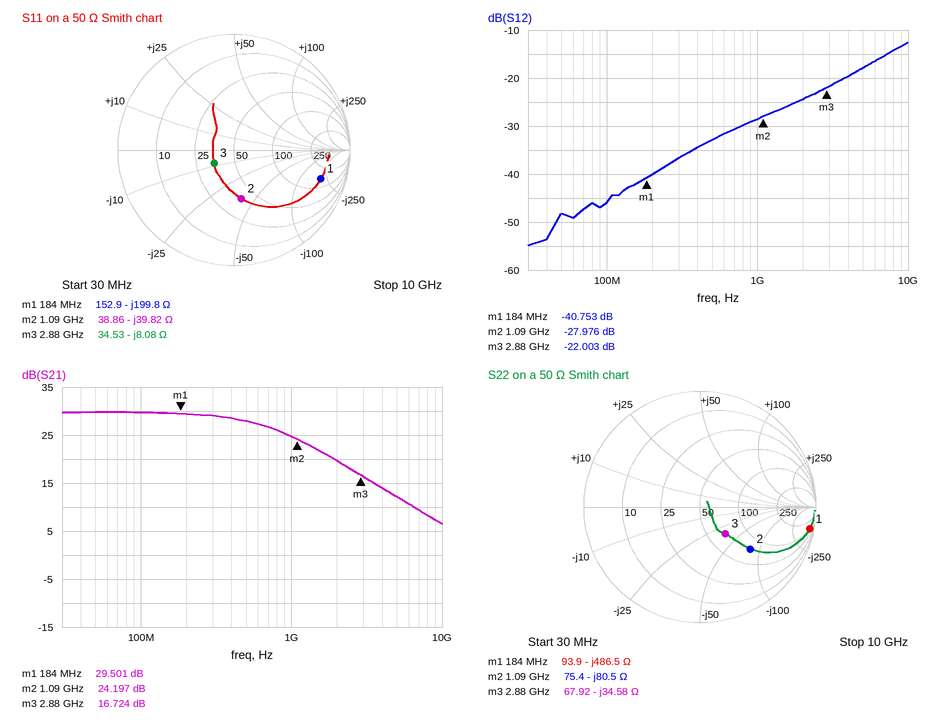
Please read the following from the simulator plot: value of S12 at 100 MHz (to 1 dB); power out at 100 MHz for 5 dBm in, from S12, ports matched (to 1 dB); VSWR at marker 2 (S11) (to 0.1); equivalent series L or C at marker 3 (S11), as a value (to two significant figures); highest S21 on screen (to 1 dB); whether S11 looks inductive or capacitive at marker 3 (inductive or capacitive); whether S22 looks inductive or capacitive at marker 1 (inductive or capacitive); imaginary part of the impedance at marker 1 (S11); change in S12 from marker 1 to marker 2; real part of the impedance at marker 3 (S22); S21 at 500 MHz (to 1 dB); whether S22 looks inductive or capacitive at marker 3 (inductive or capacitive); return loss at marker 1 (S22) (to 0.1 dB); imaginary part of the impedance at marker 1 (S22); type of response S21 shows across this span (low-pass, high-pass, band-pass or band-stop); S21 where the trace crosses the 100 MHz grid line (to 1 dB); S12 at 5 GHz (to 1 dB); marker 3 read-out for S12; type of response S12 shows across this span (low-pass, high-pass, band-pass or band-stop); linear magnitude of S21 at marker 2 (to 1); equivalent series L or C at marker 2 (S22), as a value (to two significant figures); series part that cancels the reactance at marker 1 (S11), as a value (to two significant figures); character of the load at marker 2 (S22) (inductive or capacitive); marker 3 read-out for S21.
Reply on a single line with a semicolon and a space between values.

-46 dB; -41 dBm; 2.5; 6.8 pF; 30 dB; capacitive; capacitive; -199.8 Ω; 12.777 dB; 67.92 Ω; 28 dB; capacitive; 0.3 dB; -486.5 Ω; low-pass; 30 dB; -18 dB; -22.003 dB; high-pass; 16; 1.8 pF; 170 nH; capacitive; 16.724 dB
